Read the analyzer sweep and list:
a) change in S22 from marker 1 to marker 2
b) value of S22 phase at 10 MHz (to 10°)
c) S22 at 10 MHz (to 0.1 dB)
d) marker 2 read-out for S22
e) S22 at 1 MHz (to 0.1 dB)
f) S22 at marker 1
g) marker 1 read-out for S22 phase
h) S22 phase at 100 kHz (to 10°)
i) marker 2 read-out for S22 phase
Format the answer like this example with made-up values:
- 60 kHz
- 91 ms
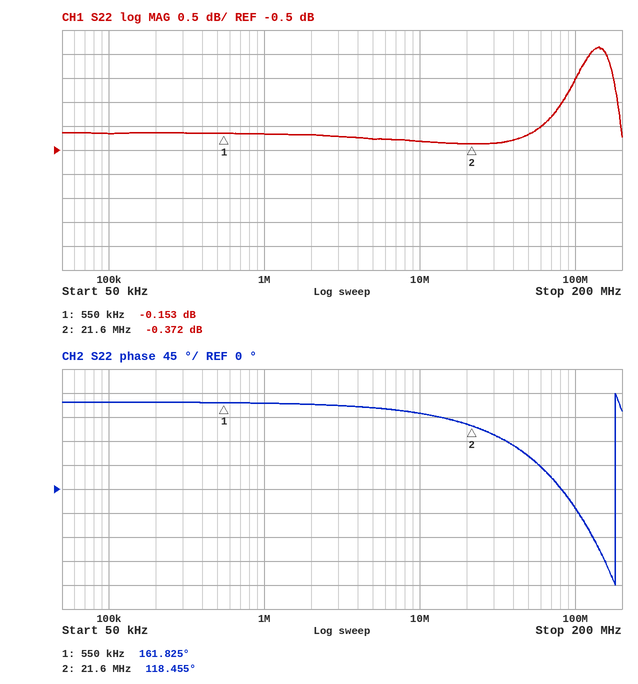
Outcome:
- -0.219 dB
- 140°
- -0.3 dB
- -0.372 dB
- -0.2 dB
- -0.153 dB
- 161.825°
- 160°
- 118.455°
